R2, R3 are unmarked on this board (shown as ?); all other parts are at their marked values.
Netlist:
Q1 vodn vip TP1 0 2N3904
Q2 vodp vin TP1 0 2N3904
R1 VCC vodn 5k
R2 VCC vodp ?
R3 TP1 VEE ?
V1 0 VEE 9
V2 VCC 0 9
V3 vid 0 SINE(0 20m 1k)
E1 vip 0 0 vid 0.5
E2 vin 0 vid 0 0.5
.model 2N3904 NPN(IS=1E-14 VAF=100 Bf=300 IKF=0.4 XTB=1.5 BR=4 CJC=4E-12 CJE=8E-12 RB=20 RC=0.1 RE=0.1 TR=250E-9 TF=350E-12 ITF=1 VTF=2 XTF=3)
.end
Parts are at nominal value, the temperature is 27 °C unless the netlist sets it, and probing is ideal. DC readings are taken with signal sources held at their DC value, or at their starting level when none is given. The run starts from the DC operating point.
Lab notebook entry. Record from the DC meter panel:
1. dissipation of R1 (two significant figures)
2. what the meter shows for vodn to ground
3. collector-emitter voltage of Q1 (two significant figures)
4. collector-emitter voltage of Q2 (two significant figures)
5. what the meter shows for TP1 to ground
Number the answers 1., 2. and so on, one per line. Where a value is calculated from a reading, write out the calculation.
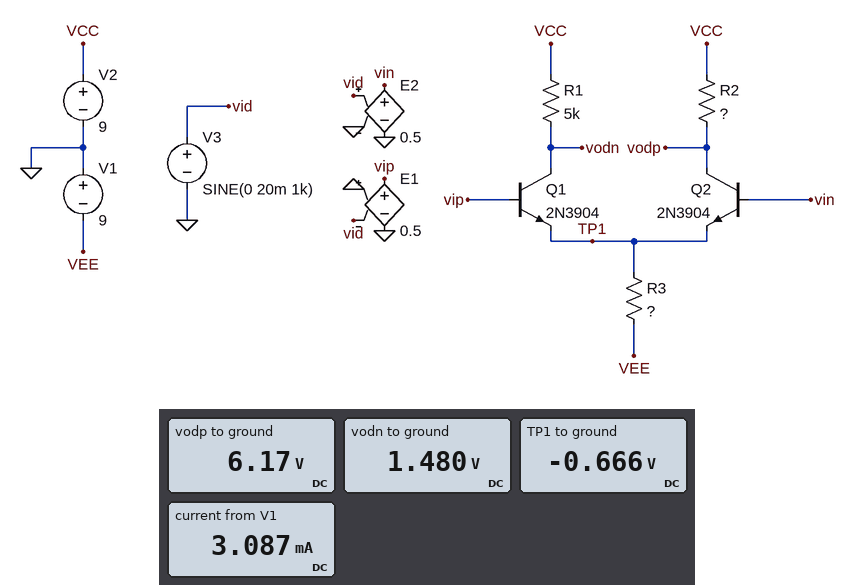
1. (9 V - 1.48 V)^2 / 5 kΩ = 11 mW
2. 1.480 V
3. 1.48 V - (-666 mV) = 2.1 V
4. 6.17 V - (-666 mV) = 6.8 V
5. -0.666 V
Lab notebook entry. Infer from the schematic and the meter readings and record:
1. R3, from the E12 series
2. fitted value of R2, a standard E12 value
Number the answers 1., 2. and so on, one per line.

1. 2.7 kΩ
2. 1.8 kΩ
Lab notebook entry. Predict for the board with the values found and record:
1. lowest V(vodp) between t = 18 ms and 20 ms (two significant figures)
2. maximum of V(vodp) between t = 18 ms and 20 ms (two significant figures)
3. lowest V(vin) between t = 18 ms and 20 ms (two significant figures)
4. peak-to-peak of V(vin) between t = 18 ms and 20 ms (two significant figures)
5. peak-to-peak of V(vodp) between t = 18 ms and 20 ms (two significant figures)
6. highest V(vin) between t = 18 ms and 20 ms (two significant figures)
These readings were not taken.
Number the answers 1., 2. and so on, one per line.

1. 5.2 V
2. 7.0 V
3. -10 mV
4. 20 mV
5. 1.8 V
6. 10 mV
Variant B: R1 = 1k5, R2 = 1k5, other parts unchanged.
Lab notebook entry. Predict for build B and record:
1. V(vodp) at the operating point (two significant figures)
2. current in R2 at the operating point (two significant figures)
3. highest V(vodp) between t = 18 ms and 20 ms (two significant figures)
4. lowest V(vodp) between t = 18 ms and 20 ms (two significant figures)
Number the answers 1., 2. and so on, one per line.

1. 6.7 V
2. 1.5 mA
3. 7.5 V
4. 5.9 V
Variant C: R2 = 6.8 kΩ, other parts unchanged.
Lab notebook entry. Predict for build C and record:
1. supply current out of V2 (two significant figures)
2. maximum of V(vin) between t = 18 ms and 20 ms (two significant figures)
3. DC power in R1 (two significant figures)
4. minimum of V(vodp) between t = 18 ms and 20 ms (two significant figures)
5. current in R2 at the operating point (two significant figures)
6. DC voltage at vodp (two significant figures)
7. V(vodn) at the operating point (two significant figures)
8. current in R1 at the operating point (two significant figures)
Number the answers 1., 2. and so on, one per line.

1. 3.0 mA
2. 10 mV
3. 13 mW
4. -650 mV
5. 1.4 mA
6. -600 mV
7. 840 mV
8. 1.6 mA
